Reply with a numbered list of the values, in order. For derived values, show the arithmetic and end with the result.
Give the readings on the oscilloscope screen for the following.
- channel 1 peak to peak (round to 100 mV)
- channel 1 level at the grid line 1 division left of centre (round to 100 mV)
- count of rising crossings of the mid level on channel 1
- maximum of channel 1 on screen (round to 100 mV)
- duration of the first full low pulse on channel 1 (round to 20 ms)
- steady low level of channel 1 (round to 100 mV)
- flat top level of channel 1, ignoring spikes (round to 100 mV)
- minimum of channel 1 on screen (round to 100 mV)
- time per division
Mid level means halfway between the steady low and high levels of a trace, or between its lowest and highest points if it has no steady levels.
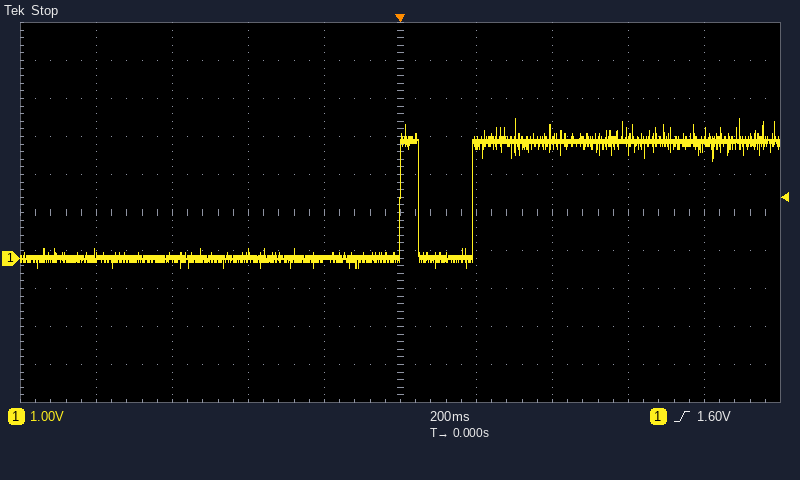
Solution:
1. 3.7 V − (-200 mV) = 3.9 V
2. 0.0 V
3. 2
4. 3.7 V
5. 140 ms
6. 0.0 V
7. 3.1 V
8. -200 mV
9. 200 ms
